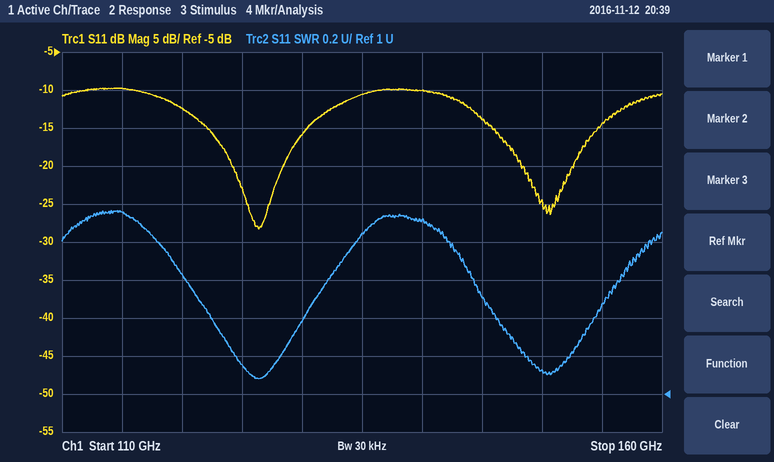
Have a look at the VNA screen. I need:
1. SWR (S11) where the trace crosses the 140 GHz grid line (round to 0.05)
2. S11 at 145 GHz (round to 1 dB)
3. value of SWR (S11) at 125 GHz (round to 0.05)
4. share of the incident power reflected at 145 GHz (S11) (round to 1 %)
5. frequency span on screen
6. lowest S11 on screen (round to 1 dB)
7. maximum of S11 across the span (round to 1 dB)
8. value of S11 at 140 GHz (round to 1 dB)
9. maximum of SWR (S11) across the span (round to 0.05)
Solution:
1.90
-14 dB
1.15
4 %
50 GHz
-28 dB
-10 dB
-10 dB
1.95
